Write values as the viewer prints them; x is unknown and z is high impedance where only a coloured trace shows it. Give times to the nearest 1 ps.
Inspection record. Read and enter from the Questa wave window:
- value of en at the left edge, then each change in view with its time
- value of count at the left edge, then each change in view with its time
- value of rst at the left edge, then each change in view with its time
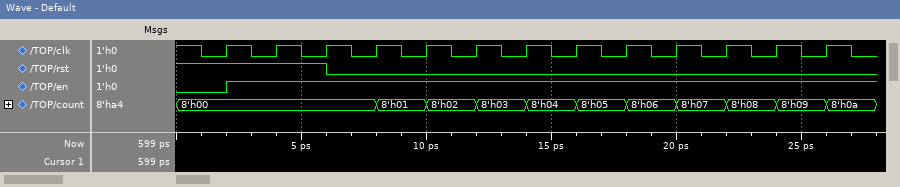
0, 1 at 2 ps
8'h00, 8'h01 at 8 ps, 8'h02 at 10 ps, 8'h03 at 12 ps, 8'h04 at 14 ps, 8'h05 at 16 ps, 8'h06 at 18 ps, 8'h07 at 20 ps, 8'h08 at 22 ps, 8'h09 at 24 ps, 8'h0a at 26 ps
1, 0 at 6 ps
